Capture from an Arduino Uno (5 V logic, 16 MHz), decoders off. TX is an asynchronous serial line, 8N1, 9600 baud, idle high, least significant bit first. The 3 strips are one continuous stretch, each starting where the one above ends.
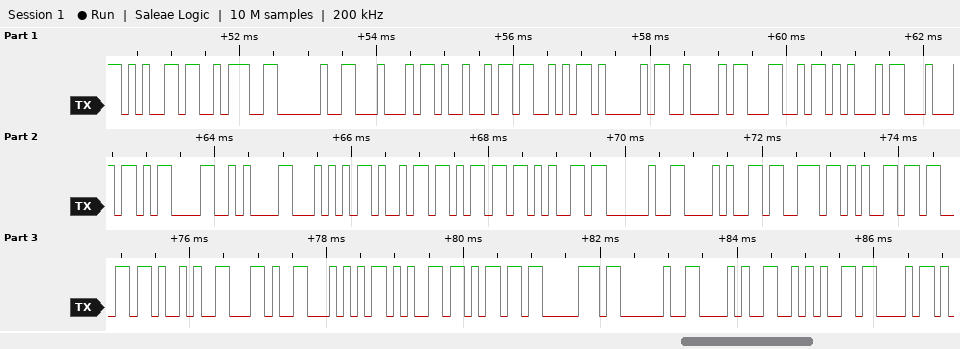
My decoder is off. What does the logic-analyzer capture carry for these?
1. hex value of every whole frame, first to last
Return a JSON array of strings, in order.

["65 3A 20 44 49 53 41 42 4C 45 44 0D 0A 54 69 6D 65 20 28 73 65 63 29 2C 54 65 6D 70 20 28 2A 43"]
